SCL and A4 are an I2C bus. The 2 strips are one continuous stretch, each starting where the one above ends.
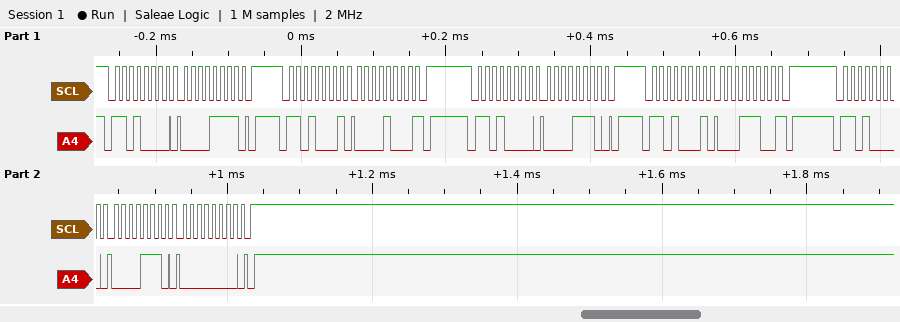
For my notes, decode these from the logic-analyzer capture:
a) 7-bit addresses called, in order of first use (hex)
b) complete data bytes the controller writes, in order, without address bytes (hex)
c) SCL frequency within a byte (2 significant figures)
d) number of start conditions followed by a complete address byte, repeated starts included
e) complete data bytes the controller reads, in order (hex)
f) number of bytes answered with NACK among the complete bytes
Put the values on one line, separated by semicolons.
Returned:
0x68; 0F 0E 0E 00; 100 kHz; 5; 08 1C; 2
